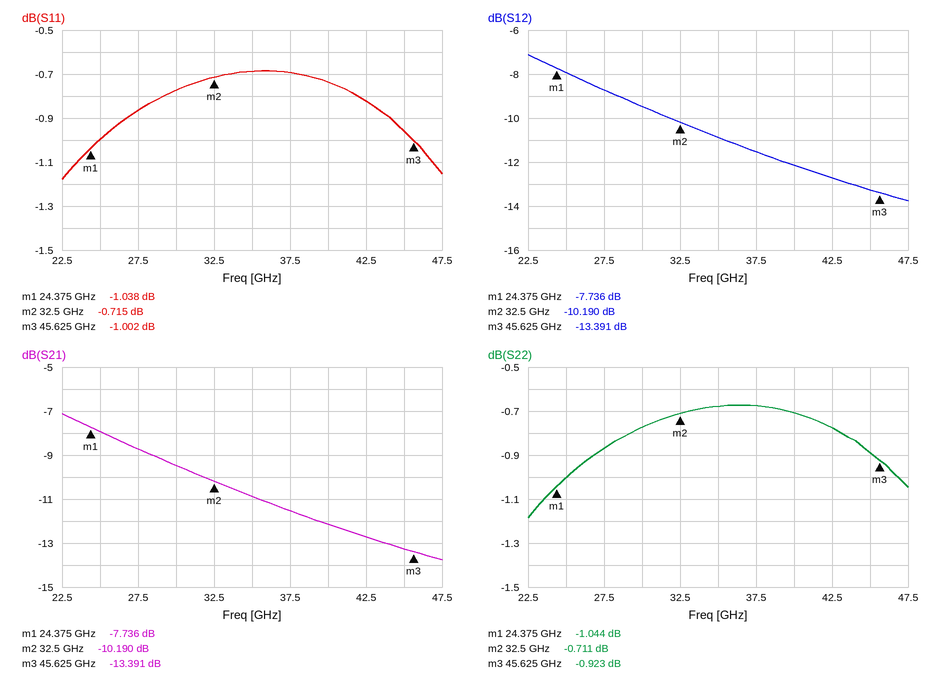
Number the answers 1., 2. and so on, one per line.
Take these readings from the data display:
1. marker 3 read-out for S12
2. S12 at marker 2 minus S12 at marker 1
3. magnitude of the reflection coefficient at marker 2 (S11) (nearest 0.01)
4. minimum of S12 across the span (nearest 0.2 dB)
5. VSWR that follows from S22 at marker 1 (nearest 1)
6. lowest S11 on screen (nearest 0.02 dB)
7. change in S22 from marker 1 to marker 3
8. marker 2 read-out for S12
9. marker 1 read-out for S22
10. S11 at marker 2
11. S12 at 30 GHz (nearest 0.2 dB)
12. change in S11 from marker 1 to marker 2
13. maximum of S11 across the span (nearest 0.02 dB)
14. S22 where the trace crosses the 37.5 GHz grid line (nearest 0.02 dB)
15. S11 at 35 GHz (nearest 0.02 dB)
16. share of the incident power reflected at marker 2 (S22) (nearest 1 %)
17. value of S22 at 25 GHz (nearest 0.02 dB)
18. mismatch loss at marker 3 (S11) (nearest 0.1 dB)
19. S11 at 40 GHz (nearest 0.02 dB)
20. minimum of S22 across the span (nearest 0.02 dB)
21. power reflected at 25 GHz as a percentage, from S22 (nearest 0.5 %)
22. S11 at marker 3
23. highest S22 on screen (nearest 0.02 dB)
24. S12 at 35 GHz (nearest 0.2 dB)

1. -13.391 dB
2. -2.454 dB
3. 0.92
4. -13.8 dB
5. 17
6. -1.18 dB
7. 0.121 dB
8. -10.190 dB
9. -1.044 dB
10. -0.715 dB
11. -9.4 dB
12. 0.323 dB
13. -0.68 dB
14. -0.68 dB
15. -0.68 dB
16. 85 %
17. -1.00 dB
18. 6.9 dB
19. -0.74 dB
20. -1.18 dB
21. 79.5 %
22. -1.002 dB
23. -0.68 dB
24. -10.8 dB
